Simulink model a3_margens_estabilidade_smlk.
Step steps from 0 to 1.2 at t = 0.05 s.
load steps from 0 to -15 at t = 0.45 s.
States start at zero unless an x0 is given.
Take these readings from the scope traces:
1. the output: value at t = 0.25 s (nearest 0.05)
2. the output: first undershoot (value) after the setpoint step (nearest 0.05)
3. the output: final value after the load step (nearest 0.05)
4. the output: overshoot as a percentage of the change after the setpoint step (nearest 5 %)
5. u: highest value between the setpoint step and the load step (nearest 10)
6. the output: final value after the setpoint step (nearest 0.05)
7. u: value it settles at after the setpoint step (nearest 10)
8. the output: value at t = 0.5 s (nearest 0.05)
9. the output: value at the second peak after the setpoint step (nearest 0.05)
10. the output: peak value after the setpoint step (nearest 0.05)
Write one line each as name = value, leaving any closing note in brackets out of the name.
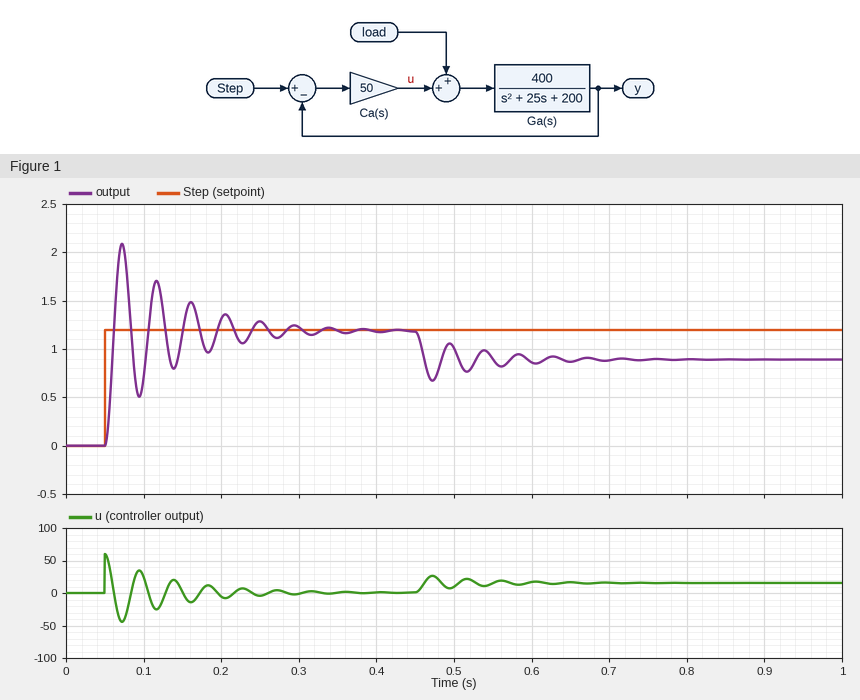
the output: value at t = 0.25 s = 1.30
the output: first undershoot (value) after the setpoint step = 0.50
the output: final value after the load step = 0.90
the output: overshoot as a percentage of the change after the setpoint step = 75 %
u: highest value between the setpoint step and the load step = 60
the output: final value after the setpoint step = 1.20
u: value it settles at after the setpoint step = 0
the output: value at t = 0.5 s = 1.00
the output: value at the second peak after the setpoint step = 1.70
the output: peak value after the setpoint step = 2.10
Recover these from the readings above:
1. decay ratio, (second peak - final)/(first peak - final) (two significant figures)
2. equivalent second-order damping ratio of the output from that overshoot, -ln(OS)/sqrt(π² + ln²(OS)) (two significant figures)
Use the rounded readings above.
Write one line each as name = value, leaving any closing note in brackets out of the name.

decay ratio, (second peak - final)/(first peak - final) = 0.56
equivalent second-order damping ratio of the output from that overshoot, -ln(OS)/sqrt(π² + ln²(OS)) = 0.091
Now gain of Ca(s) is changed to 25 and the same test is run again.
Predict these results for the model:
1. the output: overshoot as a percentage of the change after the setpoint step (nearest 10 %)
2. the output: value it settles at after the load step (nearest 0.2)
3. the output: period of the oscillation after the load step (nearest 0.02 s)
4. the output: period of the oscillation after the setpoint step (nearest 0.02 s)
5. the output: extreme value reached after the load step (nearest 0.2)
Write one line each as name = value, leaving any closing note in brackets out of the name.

the output: overshoot as a percentage of the change after the setpoint step = 70 %
the output: value it settles at after the load step = 0.6
the output: period of the oscillation after the load step = 0.06 s
the output: period of the oscillation after the setpoint step = 0.06 s
the output: extreme value reached after the load step = 0.2
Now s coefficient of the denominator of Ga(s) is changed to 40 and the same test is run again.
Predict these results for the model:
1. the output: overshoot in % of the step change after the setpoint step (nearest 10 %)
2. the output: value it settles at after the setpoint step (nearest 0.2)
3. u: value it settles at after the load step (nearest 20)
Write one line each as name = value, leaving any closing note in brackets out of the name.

the output: overshoot in % of the step change after the setpoint step = 60 %
the output: value it settles at after the setpoint step = 1.2
u: value it settles at after the load step = 20
